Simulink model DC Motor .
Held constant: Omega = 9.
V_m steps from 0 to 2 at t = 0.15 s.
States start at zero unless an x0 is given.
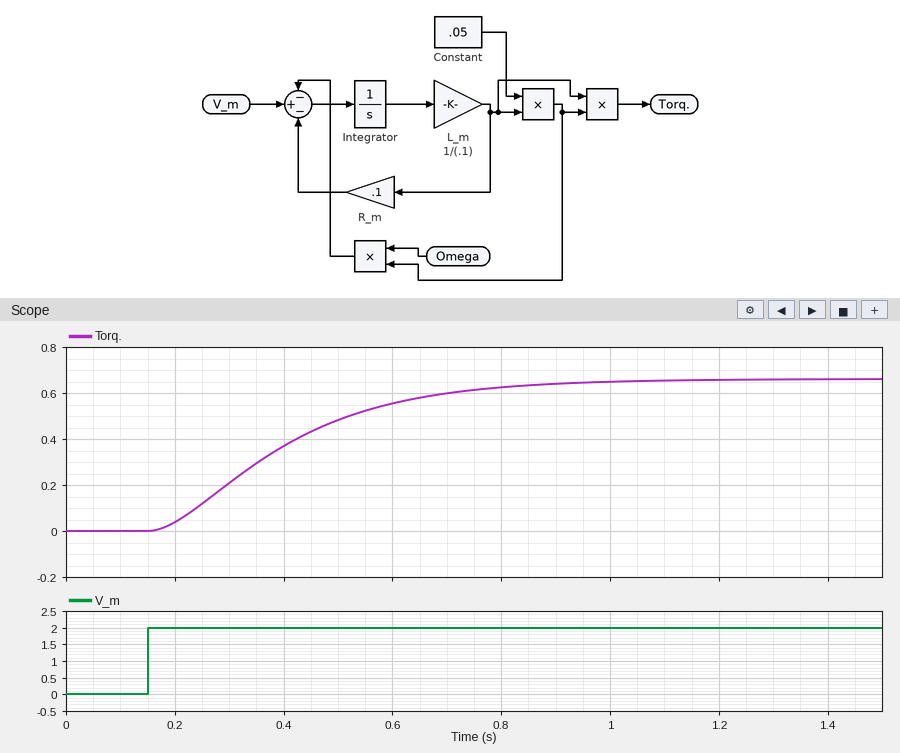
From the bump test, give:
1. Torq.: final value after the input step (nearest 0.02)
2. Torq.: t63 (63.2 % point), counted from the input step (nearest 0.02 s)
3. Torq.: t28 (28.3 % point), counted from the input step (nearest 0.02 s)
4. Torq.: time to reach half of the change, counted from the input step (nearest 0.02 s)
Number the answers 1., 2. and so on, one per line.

1. 0.66
2. 0.28 s
3. 0.14 s
4. 0.22 s
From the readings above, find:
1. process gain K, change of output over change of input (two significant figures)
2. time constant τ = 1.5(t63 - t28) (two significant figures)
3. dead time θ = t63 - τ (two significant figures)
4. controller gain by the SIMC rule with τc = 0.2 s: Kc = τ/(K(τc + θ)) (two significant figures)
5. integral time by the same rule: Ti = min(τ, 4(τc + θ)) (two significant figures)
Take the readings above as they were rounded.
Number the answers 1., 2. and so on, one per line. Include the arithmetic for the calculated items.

1. (0.66 - 0) / 2 = 0.33
2. 1.5 × (0.28 - 0.14) = 0.21 s
3. 0.28 - 0.21 = 0.070 s
4. 0.21 / (0.33 × (0.2 + 0.07)) = 2.4
5. min(0.21, 4 × (0.2 + 0.07)) = 0.21 s
